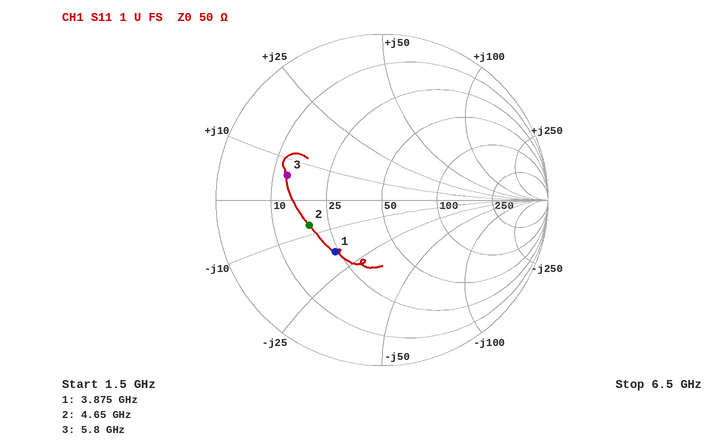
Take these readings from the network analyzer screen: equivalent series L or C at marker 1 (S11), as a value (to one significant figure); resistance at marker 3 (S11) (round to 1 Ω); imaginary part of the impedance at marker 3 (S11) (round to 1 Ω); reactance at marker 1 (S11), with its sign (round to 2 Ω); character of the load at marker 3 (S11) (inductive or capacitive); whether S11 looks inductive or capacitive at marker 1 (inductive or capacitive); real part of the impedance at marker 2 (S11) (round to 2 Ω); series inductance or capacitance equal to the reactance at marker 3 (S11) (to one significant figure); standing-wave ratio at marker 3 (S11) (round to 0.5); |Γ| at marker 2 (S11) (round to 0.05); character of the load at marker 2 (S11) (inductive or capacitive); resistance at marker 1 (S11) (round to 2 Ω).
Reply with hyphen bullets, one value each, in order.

- 2 pF
- 13 Ω
- +6 Ω
- -18 Ω
- inductive
- capacitive
- 18 Ω
- 200 pH
- 4.0
- 0.45
- capacitive
- 24 Ω
